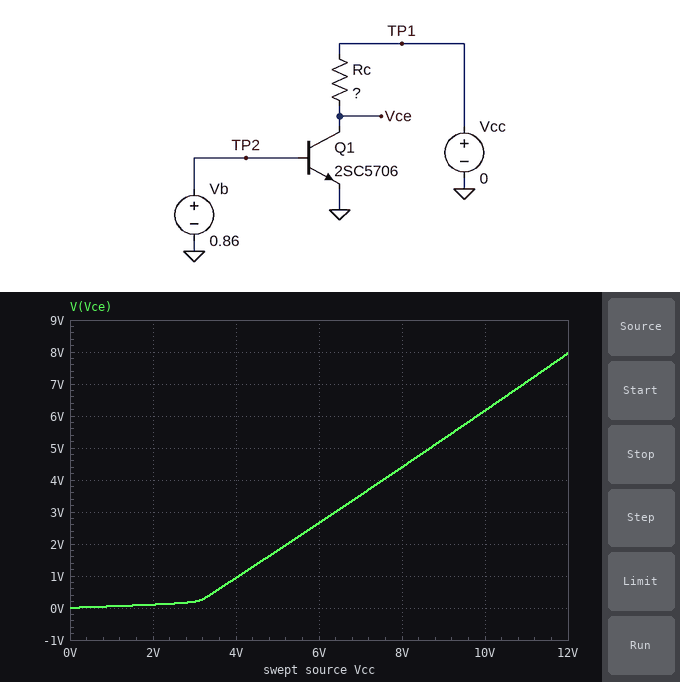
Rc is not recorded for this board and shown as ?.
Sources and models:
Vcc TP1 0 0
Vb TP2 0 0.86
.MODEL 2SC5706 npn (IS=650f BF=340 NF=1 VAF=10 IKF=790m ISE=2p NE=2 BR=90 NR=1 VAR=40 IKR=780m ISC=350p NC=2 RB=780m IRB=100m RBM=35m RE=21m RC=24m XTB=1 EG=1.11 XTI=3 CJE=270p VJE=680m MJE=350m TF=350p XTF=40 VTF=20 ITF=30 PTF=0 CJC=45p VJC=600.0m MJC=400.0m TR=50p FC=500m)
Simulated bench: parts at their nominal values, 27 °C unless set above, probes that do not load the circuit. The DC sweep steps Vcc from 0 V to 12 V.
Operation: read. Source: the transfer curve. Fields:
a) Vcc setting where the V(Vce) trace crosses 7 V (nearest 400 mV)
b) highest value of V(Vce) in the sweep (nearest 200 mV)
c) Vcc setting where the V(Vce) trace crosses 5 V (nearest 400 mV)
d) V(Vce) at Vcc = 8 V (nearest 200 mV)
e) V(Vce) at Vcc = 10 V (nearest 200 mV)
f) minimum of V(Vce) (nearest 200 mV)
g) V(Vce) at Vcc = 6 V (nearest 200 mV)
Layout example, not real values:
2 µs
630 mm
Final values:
10.8 V
8.0 V
8.8 V
4.4 V
6.2 V
0 V
2.6 V
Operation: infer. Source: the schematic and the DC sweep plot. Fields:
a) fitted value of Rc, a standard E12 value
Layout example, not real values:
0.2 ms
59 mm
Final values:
1.2 Ω
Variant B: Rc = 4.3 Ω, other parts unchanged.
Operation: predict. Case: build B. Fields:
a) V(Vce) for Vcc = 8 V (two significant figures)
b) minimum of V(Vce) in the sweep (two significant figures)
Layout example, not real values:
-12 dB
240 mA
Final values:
130 mV
5.7 mV
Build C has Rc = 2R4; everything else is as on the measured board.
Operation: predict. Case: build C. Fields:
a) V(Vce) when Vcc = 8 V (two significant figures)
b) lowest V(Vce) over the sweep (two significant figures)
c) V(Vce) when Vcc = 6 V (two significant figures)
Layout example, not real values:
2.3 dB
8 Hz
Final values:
1.6 V
5.7 mV
230 mV
